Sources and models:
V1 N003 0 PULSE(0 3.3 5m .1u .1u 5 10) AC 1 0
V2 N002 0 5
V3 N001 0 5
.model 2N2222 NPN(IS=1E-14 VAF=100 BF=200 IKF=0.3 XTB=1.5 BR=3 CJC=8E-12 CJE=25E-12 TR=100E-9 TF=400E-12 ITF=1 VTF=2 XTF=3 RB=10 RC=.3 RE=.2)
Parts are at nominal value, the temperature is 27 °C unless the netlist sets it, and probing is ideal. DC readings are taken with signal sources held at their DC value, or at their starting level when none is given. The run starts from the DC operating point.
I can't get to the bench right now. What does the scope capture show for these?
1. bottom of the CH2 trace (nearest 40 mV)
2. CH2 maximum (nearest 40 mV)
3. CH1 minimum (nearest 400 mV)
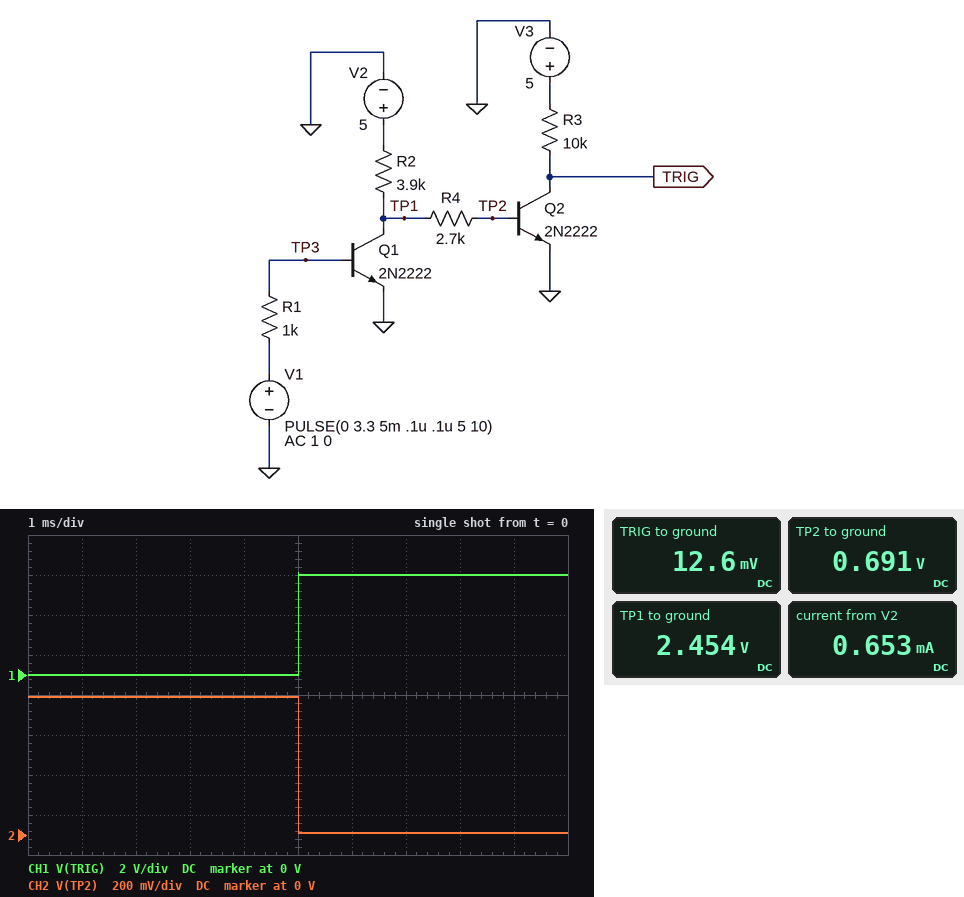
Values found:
0 V
680 mV
0 V
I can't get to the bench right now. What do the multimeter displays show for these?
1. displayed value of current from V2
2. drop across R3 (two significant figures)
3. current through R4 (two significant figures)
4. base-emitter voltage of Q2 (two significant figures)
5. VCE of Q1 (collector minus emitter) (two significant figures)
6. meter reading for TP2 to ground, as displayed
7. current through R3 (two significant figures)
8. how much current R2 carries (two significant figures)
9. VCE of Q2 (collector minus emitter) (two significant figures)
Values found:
0.653 mA
5.0 V
650 µA
690 mV
2.5 V
0.691 V
500 µA
650 µA
13 mV
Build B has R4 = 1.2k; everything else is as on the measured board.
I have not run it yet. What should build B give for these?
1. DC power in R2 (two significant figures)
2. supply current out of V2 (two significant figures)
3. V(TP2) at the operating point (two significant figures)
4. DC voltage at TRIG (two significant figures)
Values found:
2.8 mW
840 µA
700 mV
12 mV
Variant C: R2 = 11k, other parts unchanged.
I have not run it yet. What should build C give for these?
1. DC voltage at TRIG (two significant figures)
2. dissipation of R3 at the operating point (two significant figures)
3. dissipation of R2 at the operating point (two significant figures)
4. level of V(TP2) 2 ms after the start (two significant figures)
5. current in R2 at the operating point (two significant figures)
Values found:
17 mV
2.5 mW
1.1 mW
670 mV
320 µA
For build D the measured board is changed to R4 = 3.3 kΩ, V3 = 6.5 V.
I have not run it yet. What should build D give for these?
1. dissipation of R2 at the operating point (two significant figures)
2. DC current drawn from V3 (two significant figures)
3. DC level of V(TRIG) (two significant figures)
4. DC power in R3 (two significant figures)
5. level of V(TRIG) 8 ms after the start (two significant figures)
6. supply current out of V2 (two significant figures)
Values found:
1.4 mW
650 µA
14 mV
4.2 mW
6.5 V
600 µA
